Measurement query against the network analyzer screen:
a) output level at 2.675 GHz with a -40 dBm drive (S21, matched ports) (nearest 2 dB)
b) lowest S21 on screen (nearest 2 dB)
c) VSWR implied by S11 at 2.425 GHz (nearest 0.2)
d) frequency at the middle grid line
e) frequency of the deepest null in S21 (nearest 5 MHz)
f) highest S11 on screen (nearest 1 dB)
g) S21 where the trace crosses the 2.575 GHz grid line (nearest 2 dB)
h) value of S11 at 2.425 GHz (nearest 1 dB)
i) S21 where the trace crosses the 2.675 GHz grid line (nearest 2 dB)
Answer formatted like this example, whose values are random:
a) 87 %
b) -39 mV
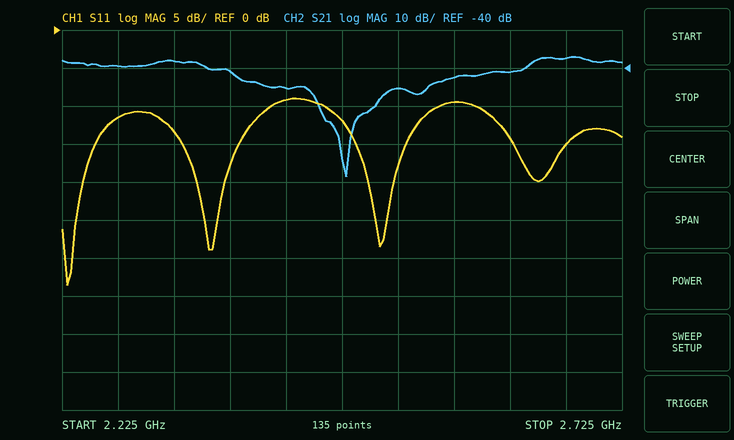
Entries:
a) -78 dBm
b) -68 dB
c) 2.0
d) 2.475 GHz
e) 2.480 GHz
f) -9 dB
g) -42 dB
h) -9 dB
i) -38 dB
